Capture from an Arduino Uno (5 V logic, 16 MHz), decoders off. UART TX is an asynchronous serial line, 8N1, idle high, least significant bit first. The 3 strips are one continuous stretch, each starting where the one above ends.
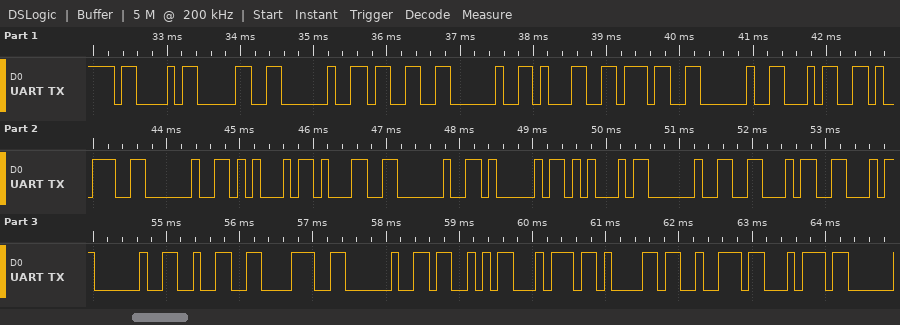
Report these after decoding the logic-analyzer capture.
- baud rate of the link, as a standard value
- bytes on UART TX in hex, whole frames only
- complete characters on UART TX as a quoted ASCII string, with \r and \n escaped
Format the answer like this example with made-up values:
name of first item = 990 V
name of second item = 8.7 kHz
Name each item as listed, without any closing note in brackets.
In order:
baud rate of the link, as a standard value = 9600 baud
bytes on UART TX in hex, whole frames only = 43 30 20 33 20 31 37 20 34 39 20 45 31 20 41 45 20 46 46 20 32 38 20 53 74 61 72 74
complete characters on UART TX as a quoted ASCII string, with \r and \n escaped = "C0 3 17 49 E1 AE FF 28 Start"
